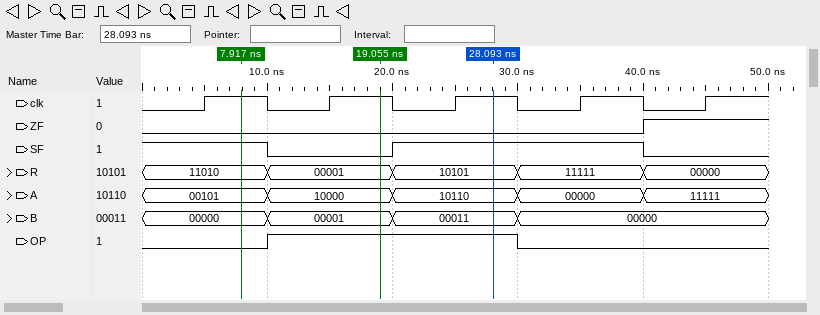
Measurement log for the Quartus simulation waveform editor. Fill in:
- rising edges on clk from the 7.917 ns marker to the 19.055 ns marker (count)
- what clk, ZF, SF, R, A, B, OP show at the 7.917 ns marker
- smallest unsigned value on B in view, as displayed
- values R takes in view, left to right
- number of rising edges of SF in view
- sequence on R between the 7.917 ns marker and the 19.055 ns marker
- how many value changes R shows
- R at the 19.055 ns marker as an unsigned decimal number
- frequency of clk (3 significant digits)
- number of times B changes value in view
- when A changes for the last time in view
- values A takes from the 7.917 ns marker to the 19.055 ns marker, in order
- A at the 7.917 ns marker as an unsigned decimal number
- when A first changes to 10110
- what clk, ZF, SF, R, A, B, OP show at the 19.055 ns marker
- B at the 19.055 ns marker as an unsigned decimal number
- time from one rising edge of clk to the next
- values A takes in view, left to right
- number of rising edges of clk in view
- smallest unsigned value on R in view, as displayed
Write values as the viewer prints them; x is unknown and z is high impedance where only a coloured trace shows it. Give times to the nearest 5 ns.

1
clk=1, ZF=0, SF=1, R=11010, A=00101, B=00000, OP=0
00000
11010, 00001, 10101, 11111, 00000
1
11010, 00001
4
1
100 MHz
3
40 ns
00101, 10000
5
20 ns
clk=1, ZF=0, SF=0, R=00001, A=10000, B=00001, OP=1
1
10 ns
00101, 10000, 10110, 00000, 11111
5
00000
